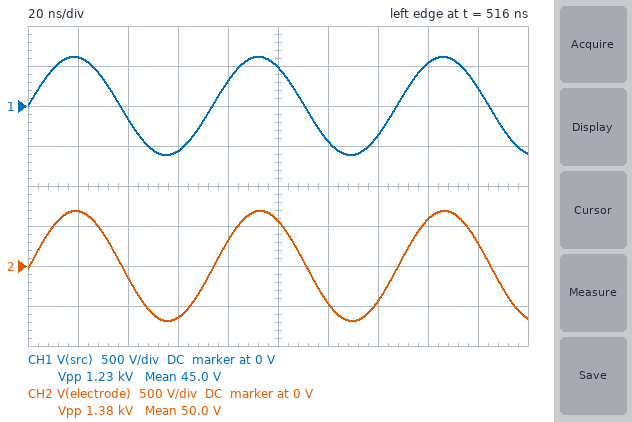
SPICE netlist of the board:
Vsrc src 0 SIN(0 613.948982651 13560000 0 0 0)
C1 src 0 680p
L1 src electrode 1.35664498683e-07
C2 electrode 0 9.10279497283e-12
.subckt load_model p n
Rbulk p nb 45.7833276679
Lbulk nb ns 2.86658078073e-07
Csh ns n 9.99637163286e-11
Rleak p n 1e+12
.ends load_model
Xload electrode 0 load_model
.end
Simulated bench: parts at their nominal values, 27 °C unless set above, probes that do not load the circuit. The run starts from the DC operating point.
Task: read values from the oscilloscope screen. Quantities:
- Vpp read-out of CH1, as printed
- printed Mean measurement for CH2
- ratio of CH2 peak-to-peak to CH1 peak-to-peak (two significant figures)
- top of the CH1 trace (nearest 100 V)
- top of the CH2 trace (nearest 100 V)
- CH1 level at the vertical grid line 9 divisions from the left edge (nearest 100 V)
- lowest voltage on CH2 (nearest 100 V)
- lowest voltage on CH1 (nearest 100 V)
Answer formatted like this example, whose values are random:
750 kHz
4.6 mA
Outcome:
1.23 kV
50.0 V
1.1
600 V
700 V
200 V
-700 V
-600 V
